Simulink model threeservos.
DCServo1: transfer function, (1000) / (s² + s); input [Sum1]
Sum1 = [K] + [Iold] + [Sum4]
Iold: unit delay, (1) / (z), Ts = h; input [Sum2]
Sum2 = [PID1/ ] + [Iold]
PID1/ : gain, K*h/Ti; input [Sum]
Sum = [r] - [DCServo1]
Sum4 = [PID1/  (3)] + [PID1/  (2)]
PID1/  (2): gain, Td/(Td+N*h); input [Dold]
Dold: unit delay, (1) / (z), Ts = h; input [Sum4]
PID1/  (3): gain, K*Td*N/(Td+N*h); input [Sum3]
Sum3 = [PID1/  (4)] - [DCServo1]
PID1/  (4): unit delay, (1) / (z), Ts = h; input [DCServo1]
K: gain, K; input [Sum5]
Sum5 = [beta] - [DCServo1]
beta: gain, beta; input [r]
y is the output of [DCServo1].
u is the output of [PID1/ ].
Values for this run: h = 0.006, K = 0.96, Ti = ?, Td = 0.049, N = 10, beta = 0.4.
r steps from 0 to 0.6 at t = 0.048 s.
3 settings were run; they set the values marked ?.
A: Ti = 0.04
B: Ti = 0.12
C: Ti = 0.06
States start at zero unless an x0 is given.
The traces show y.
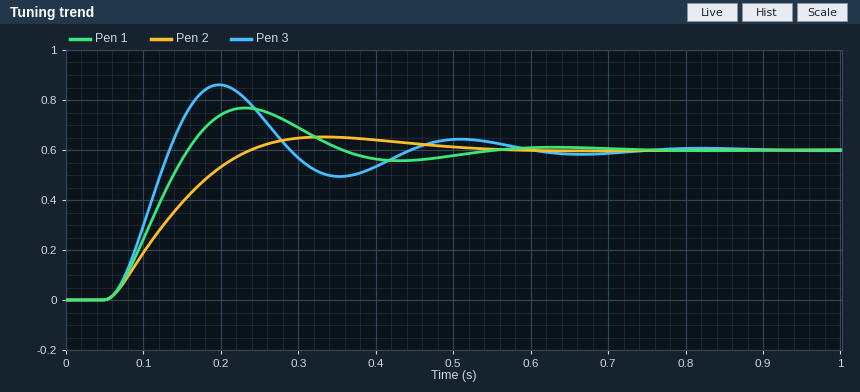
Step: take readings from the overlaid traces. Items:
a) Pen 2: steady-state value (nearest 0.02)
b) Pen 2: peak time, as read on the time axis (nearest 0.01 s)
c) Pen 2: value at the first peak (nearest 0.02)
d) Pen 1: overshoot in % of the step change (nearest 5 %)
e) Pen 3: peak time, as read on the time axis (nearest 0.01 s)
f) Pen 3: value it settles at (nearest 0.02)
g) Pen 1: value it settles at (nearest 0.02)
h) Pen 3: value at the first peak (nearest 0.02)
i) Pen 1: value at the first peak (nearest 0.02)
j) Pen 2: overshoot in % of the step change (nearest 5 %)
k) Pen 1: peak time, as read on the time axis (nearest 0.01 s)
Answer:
0.60
0.33 s
0.66
30 %
0.20 s
0.60
0.60
0.86
0.76
10 %
0.23 s
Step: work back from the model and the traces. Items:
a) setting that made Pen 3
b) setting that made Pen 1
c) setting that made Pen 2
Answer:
A
C
B
